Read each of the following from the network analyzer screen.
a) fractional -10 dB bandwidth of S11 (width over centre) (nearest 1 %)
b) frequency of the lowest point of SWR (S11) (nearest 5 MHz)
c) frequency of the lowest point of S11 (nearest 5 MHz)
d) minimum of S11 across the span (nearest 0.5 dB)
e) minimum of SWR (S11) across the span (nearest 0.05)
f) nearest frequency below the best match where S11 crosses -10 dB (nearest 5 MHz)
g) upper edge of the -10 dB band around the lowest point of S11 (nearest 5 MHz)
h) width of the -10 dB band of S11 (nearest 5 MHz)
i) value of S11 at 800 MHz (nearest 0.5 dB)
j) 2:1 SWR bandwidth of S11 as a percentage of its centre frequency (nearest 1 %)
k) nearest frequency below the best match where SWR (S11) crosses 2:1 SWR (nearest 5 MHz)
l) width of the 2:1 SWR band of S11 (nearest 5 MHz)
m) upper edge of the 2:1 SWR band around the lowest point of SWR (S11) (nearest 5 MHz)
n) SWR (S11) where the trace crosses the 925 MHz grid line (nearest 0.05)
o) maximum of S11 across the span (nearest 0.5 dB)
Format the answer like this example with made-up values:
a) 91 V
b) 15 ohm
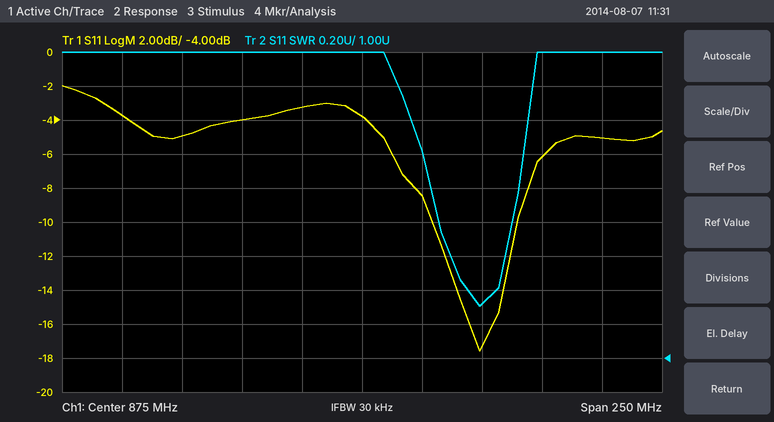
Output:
a) 4 %
b) 925 MHz
c) 925 MHz
d) -17.5 dB
e) 1.30
f) 905 MHz
g) 940 MHz
h) 35 MHz
i) -5.0 dB
j) 4 %
k) 905 MHz
l) 35 MHz
m) 940 MHz
n) 1.30
o) -2.0 dB
